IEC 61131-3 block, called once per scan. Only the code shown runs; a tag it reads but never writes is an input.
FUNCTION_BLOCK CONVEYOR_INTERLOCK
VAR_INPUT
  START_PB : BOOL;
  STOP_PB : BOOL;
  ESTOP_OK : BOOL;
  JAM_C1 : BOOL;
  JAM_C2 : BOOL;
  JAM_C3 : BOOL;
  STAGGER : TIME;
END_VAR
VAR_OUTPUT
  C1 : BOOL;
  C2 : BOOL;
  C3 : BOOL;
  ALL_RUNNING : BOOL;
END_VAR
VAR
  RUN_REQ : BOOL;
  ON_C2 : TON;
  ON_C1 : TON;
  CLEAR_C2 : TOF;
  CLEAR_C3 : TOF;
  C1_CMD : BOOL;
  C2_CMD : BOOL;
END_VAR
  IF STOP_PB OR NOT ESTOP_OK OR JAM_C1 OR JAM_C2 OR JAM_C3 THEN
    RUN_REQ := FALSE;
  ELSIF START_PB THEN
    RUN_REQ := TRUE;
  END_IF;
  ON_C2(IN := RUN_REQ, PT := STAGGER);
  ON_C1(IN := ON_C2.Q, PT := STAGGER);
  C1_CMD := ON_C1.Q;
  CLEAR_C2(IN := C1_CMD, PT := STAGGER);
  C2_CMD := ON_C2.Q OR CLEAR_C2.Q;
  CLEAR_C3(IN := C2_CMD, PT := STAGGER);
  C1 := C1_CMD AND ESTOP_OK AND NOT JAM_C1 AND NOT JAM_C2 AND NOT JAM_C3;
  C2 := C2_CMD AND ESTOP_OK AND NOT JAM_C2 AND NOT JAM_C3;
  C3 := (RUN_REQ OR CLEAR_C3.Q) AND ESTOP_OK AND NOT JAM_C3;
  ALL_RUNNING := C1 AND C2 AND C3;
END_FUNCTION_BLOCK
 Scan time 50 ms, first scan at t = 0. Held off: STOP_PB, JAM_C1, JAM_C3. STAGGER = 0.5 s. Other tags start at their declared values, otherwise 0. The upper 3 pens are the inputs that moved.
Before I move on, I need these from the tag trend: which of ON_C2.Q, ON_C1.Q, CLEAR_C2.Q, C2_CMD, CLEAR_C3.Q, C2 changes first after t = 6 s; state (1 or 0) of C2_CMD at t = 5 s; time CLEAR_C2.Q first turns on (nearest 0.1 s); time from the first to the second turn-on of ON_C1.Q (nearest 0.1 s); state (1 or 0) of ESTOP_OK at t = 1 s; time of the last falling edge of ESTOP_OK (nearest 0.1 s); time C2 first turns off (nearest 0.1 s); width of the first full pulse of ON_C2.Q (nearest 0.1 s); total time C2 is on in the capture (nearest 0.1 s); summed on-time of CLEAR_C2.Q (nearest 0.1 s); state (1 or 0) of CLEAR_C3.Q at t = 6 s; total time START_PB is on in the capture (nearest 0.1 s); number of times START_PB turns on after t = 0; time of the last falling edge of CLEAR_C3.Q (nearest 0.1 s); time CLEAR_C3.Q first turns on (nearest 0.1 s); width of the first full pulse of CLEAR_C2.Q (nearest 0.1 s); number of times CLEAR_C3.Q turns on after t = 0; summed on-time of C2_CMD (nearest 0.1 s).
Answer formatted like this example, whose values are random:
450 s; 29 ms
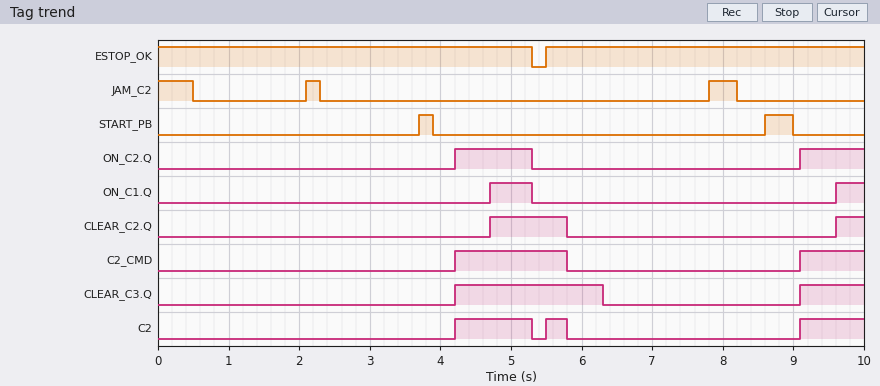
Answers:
CLEAR_C3.Q; 1; 4.7 s; 4.9 s; 1; 5.3 s; 5.3 s; 1.1 s; 2.3 s; 1.5 s; 1; 0.6 s; 2; 6.3 s; 4.2 s; 1.1 s; 2; 2.5 s
